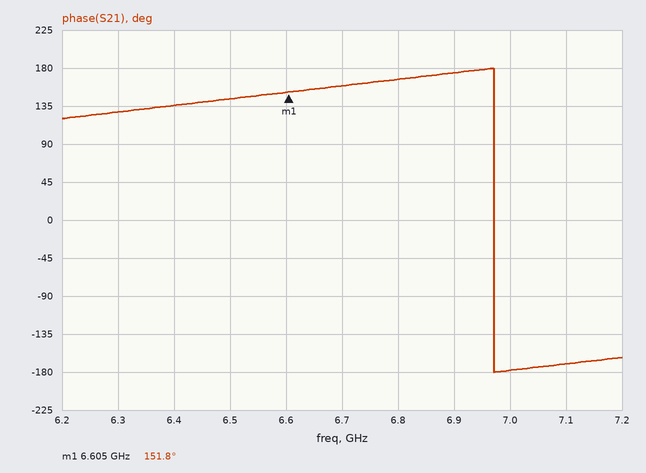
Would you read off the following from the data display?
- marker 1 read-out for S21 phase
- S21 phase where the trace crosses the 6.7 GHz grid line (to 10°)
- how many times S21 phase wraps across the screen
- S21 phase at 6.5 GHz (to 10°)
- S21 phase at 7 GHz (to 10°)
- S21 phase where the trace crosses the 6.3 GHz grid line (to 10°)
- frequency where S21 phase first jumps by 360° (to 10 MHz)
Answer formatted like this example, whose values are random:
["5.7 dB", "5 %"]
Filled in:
["151.8°", "160°", "1", "140°", "-180°", "130°", "6.97 GHz"]
